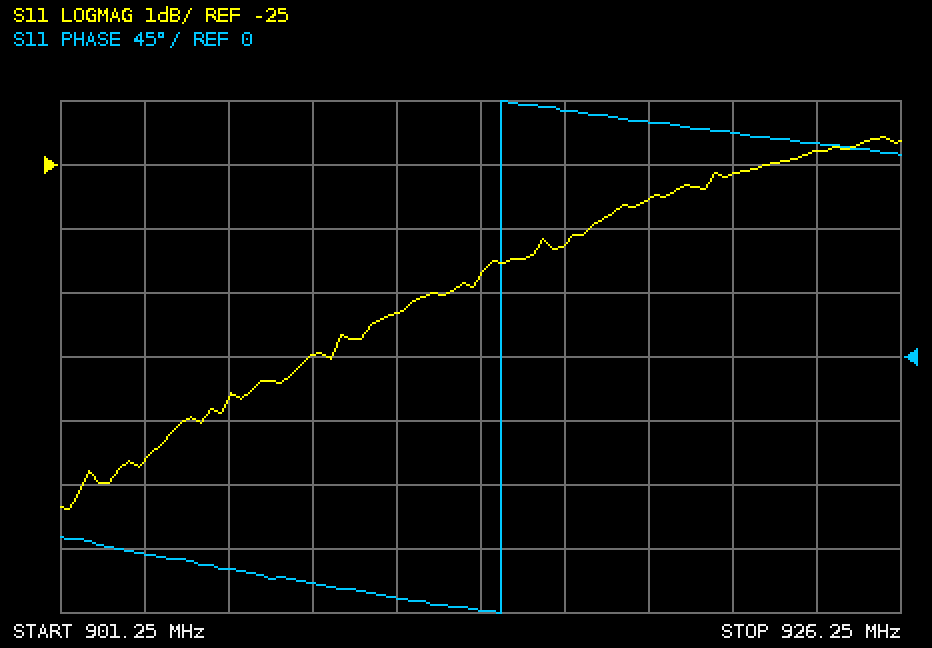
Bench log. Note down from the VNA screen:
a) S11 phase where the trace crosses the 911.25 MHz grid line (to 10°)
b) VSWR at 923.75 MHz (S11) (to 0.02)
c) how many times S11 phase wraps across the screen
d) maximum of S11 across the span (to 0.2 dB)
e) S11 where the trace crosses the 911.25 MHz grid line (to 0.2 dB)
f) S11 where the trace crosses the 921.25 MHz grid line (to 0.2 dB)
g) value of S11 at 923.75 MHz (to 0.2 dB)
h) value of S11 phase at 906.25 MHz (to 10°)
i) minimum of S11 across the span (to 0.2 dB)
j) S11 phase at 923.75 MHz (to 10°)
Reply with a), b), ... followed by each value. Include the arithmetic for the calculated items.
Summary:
a) -170°
b) |Γ| = 10^(-24.8/20) = 0.0575; VSWR = (1 + 0.0575)/(1 − 0.0575) ≈ 1.12
c) 1
d) -24.6 dB
e) -27.4 dB
f) -25.2 dB
g) -24.8 dB
h) -150°
i) -30.4 dB
j) 150°
